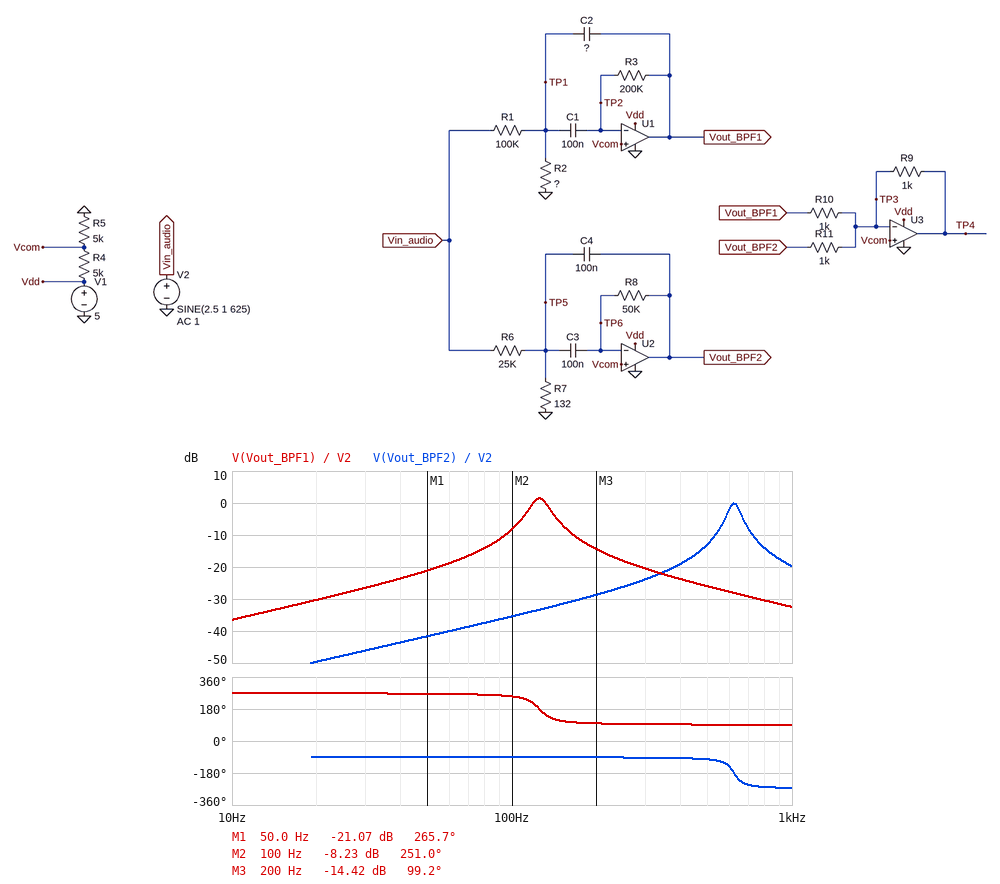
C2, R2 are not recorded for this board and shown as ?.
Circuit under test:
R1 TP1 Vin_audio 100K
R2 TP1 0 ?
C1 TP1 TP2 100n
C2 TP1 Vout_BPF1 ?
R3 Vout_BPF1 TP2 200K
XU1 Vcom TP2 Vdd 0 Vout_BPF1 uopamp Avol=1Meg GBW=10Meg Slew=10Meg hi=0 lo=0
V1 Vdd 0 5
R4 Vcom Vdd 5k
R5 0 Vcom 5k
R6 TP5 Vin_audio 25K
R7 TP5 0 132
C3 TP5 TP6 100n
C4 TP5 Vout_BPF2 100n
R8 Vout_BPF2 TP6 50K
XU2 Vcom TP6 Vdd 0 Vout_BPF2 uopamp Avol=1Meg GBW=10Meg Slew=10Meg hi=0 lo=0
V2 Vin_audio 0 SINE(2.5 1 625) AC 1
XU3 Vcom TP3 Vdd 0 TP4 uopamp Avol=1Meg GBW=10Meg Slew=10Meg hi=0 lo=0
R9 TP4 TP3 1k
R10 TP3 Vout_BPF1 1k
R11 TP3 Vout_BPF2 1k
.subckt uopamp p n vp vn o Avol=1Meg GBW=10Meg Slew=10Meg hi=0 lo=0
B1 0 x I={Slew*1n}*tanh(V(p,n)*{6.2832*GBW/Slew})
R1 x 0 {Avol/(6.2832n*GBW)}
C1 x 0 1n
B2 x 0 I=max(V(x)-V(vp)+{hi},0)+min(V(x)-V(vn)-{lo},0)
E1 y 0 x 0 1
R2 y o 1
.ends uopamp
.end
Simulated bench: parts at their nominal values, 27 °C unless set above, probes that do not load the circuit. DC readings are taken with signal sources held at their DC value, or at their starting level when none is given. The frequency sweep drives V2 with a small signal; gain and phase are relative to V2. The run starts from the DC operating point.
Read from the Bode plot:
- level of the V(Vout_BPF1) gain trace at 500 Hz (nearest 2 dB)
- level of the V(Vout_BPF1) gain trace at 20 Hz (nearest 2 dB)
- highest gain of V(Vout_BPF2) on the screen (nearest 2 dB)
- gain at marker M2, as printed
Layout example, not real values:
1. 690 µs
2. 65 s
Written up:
1. -26 dB
2. -30 dB
3. 0 dB
4. -8.23 dB
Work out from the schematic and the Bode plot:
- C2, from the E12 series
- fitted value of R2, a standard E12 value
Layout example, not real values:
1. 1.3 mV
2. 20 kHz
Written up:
1. 68 nF
2. 1.2 kΩ
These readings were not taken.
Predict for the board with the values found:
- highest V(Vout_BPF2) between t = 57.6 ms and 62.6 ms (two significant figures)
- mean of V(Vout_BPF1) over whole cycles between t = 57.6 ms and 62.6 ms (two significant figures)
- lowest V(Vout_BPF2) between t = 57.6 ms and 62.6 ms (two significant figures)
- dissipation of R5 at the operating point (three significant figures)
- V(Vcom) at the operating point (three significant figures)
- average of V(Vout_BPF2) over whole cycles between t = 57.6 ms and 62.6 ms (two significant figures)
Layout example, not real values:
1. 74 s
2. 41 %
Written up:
1. 3.5 V
2. 2.5 V
3. 1.5 V
4. 1.25 mW
5. 2.50 V
6. 2.5 V
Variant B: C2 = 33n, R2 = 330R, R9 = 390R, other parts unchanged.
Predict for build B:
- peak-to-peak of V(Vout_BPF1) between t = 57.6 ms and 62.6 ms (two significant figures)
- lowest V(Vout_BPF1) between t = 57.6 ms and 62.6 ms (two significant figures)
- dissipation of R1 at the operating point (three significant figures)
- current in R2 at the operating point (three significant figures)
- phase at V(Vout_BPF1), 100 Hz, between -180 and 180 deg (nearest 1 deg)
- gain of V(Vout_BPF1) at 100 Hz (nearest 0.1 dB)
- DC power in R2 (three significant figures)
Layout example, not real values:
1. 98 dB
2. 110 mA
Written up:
1. 220 mV
2. 2.4 V
3. 62.1 µW
4. 24.9 µA
5. -92 deg
6. -26.9 dB
7. 205 nW
